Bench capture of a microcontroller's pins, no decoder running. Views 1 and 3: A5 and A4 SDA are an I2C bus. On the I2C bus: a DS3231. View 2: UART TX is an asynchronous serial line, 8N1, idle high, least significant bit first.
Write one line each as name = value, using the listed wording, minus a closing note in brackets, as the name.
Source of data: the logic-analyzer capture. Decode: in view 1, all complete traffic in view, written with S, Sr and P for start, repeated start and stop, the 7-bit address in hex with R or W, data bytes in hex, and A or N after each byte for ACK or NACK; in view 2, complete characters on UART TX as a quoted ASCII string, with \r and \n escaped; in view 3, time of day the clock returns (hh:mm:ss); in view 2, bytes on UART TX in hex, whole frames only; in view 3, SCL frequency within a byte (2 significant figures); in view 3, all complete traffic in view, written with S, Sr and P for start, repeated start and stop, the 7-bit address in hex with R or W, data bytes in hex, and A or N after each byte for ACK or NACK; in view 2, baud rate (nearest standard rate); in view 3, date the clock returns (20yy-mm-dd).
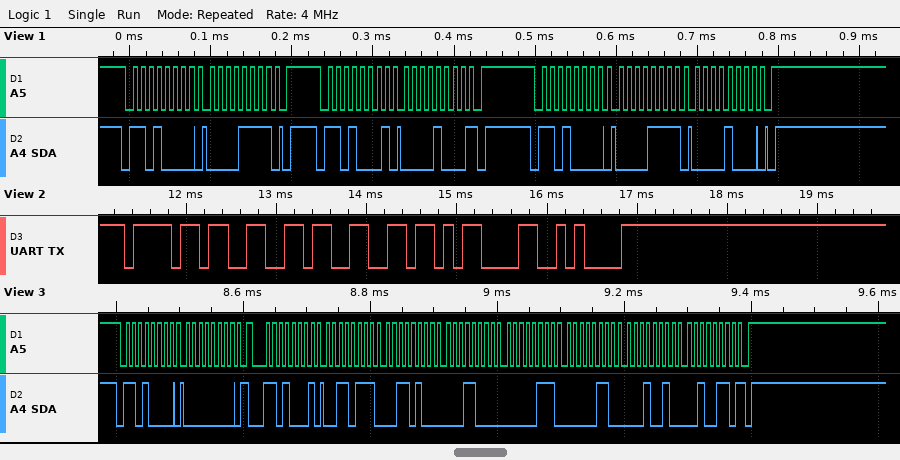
in view 1, all complete traffic in view, written with S, Sr and P for start, repeated start and stop, the 7-bit address in hex with R or W, data bytes in hex, and A or N after each byte for ACK or NACK = S 68W A 0F A P S 68R A 08 N P S 68W A 0F A 08 A P
in view 2, complete characters on UART TX as a quoted ASCII string, with \r and \n escaped = "off\r\n"
in view 3, time of day the clock returns = 18:34:37
in view 2, bytes on UART TX in hex, whole frames only = 0x6F 0x66 0x66 0x0D 0x0A
in view 3, SCL frequency within a byte = 100 kHz
in view 3, all complete traffic in view, written with S, Sr and P for start, repeated start and stop, the 7-bit address in hex with R or W, data bytes in hex, and A or N after each byte for ACK or NACK = S 68W A 00 A Sr 68R A 37 A 34 A 18 A 07 A 06 A 12 A 26 N P
in view 2, baud rate = 9600 baud
in view 3, date the clock returns = 2026-12-06
